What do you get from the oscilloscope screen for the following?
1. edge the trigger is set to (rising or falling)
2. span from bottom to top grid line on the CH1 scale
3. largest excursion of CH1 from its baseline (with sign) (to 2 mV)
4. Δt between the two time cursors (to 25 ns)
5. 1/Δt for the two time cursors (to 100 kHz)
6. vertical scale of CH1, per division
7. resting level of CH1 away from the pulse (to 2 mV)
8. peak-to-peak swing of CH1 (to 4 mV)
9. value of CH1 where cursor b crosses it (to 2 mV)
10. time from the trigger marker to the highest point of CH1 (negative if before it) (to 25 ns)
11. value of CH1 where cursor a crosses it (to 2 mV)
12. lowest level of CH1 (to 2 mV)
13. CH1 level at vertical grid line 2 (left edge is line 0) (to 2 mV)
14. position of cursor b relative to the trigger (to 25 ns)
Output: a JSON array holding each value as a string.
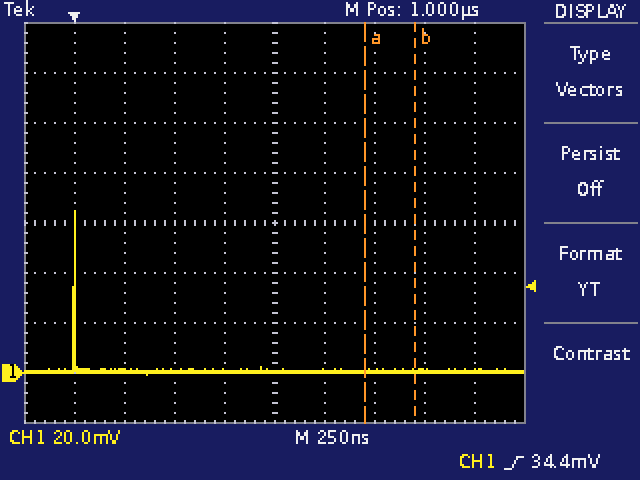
["rising", "160 mV", "+64 mV", "250 ns", "4.0 MHz", "20 mV", "0 mV", "64 mV", "0 mV", "0 ns", "0 mV", "0 mV", "0 mV", "+1.700 µs"]
